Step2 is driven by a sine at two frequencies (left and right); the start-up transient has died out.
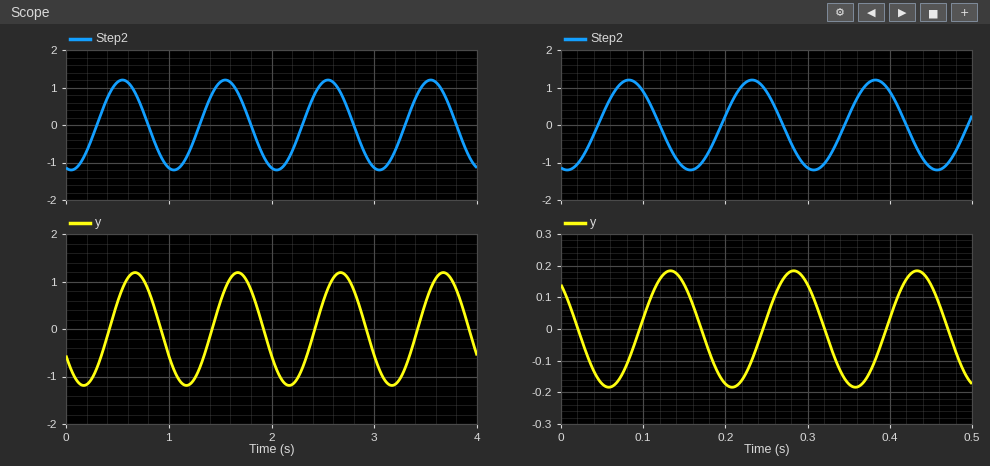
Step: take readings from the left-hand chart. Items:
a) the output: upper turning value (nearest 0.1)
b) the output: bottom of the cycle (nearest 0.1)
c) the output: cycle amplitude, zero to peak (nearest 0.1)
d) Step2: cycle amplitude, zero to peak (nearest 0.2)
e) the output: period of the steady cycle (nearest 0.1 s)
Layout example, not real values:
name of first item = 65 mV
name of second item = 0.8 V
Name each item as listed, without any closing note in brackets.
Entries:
the output: upper turning value = 1.2
the output: bottom of the cycle = -1.2
the output: cycle amplitude, zero to peak = 1.2
Step2: cycle amplitude, zero to peak = 1.2
the output: period of the steady cycle = 1.0 s
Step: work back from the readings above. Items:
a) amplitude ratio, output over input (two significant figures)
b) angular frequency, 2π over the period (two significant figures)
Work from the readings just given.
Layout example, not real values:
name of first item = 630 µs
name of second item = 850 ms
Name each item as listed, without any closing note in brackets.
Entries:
amplitude ratio, output over input = 1.0
angular frequency, 2π over the period = 6.3 rad/s
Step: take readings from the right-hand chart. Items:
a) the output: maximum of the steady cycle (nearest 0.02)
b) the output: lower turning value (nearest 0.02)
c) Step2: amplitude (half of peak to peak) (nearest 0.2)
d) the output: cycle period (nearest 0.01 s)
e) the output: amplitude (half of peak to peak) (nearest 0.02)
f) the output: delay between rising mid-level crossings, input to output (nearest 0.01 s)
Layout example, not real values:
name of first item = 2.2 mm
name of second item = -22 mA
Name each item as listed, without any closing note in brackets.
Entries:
the output: maximum of the steady cycle = 0.18
the output: lower turning value = -0.18
Step2: amplitude (half of peak to peak) = 1.2
the output: cycle period = 0.15 s
the output: amplitude (half of peak to peak) = 0.18
the output: delay between rising mid-level crossings, input to output = 0.05 s
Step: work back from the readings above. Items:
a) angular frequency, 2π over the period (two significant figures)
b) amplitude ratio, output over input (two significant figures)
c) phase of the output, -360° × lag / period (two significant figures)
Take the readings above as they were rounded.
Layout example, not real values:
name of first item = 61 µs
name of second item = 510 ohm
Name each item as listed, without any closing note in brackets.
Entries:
angular frequency, 2π over the period = 42 rad/s
amplitude ratio, output over input = 0.15
phase of the output, -360° × lag / period = -120°
